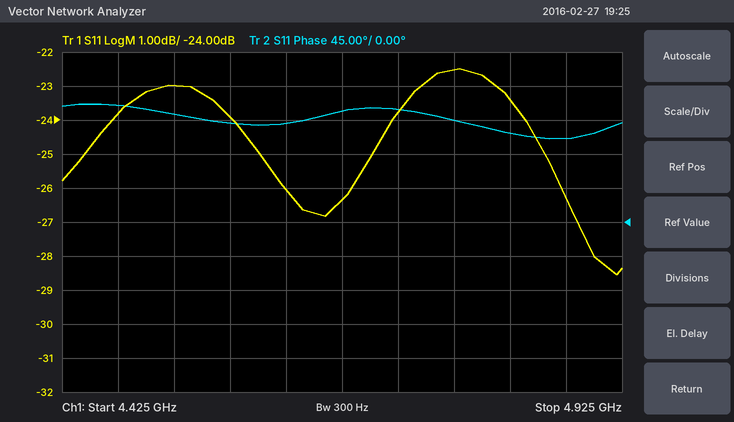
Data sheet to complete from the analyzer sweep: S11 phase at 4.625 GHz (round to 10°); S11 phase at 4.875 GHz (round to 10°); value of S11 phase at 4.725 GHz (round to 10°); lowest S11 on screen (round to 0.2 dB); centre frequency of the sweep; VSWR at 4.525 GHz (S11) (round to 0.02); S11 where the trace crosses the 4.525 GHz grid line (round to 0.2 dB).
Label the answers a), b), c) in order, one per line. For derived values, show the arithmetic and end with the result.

a) 130°
b) 110°
c) 150°
d) -28.6 dB
e) 4.675 GHz
f) |Γ| = 10^(-23/20) = 0.0708; VSWR = (1 + 0.0708)/(1 − 0.0708) ≈ 1.15, so 1.16 to the nearest 0.02
g) -23.0 dB
